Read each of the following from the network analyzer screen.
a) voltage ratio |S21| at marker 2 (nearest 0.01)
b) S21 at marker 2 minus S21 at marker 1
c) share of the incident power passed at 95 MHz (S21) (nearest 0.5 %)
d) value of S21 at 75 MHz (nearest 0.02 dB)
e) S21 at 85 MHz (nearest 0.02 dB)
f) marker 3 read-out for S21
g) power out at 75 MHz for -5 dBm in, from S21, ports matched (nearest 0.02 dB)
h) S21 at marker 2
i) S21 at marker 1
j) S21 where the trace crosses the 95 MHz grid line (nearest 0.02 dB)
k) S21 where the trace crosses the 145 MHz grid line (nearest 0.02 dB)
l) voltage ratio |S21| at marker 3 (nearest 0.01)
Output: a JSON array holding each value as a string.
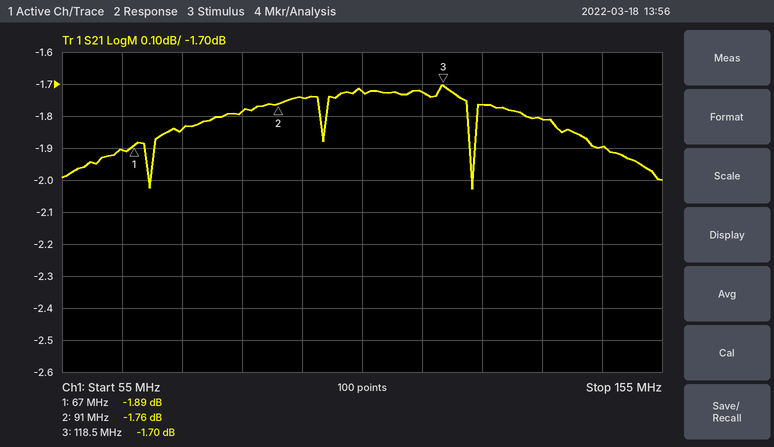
["0.82", "0.13 dB", "67.0 %", "-1.84 dB", "-1.78 dB", "-1.70 dB", "-6.84 dBm", "-1.76 dB", "-1.89 dB", "-1.74 dB", "-1.90 dB", "0.82"]
